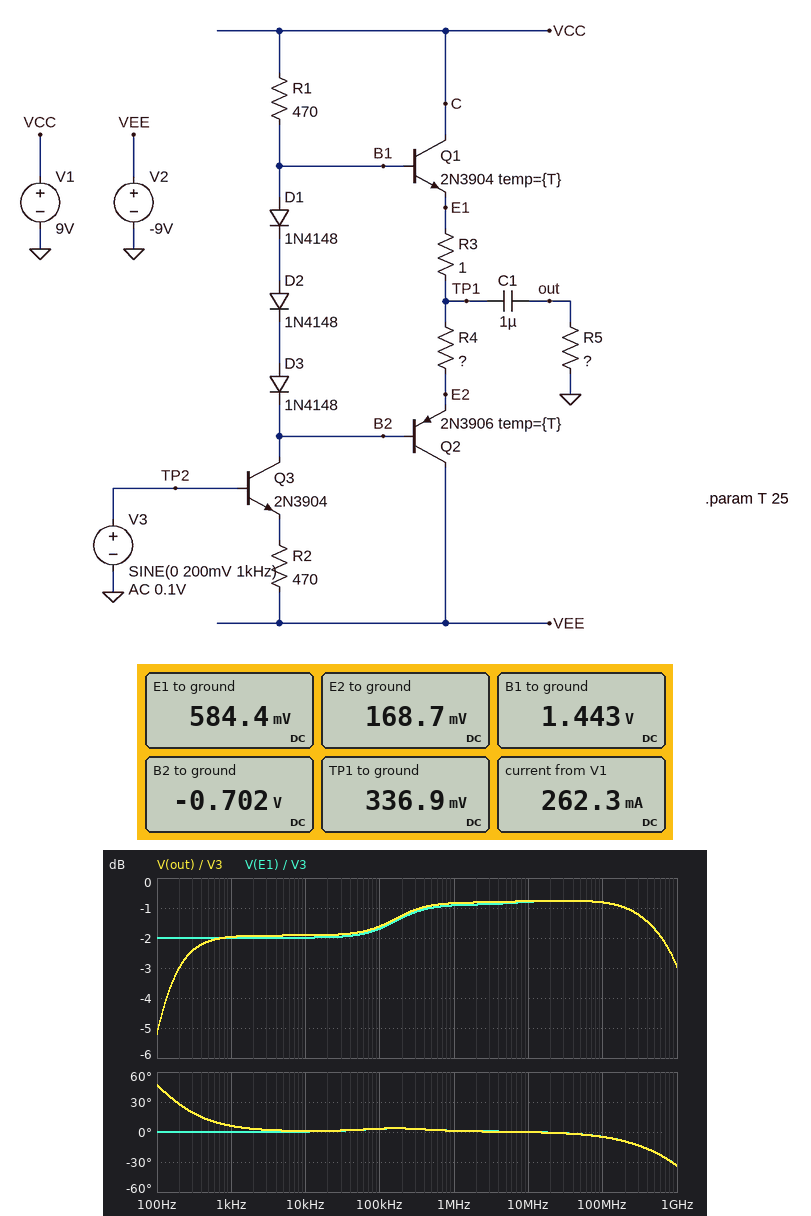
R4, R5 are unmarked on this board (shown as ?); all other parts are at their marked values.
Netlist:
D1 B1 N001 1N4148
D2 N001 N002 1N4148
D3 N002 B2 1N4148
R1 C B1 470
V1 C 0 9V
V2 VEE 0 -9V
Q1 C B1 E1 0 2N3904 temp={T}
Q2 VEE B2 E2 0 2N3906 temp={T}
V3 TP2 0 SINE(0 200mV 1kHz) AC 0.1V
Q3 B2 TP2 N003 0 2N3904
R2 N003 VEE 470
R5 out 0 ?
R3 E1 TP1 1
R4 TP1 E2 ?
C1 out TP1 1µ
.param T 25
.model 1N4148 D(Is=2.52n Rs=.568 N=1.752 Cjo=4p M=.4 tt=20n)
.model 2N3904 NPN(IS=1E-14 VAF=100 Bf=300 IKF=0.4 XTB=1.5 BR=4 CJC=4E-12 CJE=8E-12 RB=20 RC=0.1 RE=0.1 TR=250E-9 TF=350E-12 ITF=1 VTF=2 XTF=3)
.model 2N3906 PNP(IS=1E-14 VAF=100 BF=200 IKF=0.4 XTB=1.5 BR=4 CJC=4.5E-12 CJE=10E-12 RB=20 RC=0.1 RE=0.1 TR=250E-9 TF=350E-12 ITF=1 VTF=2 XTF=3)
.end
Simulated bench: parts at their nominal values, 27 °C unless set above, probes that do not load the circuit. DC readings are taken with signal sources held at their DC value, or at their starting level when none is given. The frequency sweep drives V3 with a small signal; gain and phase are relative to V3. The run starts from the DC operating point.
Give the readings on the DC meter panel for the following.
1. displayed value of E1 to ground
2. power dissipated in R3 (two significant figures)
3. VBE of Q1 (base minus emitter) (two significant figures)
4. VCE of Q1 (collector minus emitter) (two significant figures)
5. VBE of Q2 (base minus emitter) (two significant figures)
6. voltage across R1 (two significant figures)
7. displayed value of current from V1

584.4 mV
61 mW
860 mV
8.4 V
-870 mV
7.6 V
262.3 mA
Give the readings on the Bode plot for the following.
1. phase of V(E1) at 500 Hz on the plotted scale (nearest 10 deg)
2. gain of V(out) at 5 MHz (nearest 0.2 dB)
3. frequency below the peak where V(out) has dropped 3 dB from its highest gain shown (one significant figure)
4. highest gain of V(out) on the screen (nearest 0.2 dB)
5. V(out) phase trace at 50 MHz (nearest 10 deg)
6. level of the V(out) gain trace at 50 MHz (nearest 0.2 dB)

0 deg
-0.8 dB
100 Hz
-0.8 dB
0 deg
-0.8 dB
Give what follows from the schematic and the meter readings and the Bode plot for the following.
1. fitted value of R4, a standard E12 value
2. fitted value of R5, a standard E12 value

0.68 Ω
1.5 kΩ
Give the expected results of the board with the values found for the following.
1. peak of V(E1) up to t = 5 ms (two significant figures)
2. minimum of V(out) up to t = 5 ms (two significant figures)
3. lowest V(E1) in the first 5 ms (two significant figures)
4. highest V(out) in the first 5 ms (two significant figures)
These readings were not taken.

750 mV
-150 mV
450 mV
160 mV
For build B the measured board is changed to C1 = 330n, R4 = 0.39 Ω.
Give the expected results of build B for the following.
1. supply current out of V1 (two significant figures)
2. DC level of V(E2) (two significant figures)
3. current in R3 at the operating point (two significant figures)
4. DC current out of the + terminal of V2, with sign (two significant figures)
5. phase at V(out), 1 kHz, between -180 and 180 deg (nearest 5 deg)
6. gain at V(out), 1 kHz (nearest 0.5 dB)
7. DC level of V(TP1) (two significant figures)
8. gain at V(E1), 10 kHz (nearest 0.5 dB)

290 mA
190 mV
280 mA
-290 mA
20 deg
-2.5 dB
300 mV
-2.0 dB
